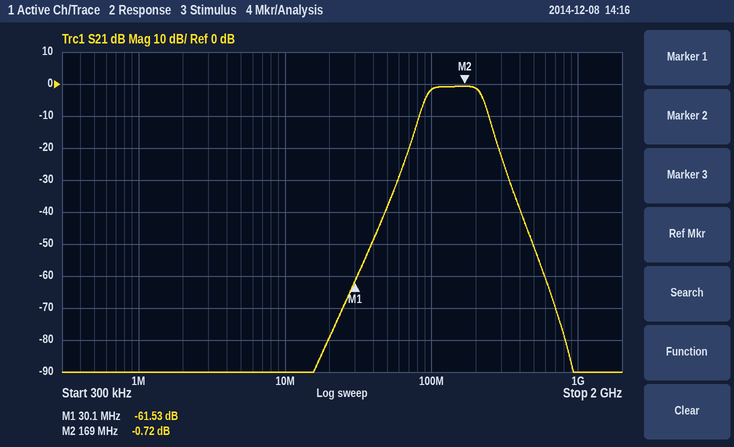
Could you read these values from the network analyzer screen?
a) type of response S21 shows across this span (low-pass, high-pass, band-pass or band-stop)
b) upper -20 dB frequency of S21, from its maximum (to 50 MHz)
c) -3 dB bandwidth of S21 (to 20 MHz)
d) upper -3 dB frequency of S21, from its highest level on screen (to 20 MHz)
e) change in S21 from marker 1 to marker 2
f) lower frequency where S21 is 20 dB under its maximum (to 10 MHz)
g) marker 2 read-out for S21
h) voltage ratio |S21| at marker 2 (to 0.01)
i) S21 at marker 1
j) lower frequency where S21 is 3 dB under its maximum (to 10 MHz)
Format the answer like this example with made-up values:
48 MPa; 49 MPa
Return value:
band-pass; 300 MHz; 120 MHz; 220 MHz; 60.81 dB; 70 MHz; -0.72 dB; 0.92; -61.53 dB; 90 MHz
